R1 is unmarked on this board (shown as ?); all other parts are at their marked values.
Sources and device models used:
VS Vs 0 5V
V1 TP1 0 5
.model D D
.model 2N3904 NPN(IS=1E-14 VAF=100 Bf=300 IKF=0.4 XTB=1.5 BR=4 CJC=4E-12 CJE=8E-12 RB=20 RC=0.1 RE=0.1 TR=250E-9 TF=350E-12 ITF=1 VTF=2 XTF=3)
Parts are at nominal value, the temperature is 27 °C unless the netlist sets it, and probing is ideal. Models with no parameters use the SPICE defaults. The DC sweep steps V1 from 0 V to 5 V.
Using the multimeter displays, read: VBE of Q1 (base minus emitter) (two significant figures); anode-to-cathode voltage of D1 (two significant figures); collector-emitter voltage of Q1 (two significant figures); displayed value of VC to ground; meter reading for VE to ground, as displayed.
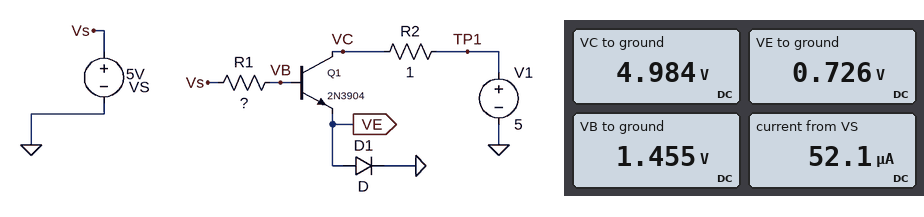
730 mV
730 mV
4.3 V
4.984 V
0.726 V
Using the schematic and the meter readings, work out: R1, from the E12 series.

68 kΩ
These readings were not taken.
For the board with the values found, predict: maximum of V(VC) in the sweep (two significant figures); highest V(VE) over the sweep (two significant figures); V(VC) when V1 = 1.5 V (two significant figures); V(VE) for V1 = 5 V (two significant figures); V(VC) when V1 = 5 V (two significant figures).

5.0 V
730 mV
1.5 V
730 mV
5.0 V
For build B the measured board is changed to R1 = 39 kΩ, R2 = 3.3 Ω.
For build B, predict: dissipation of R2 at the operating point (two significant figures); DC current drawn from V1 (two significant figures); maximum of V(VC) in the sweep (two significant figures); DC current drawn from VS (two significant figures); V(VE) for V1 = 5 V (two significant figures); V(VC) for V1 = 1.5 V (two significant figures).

2.3 mW
26 mA
4.9 V
90 µA
740 mV
1.4 V
